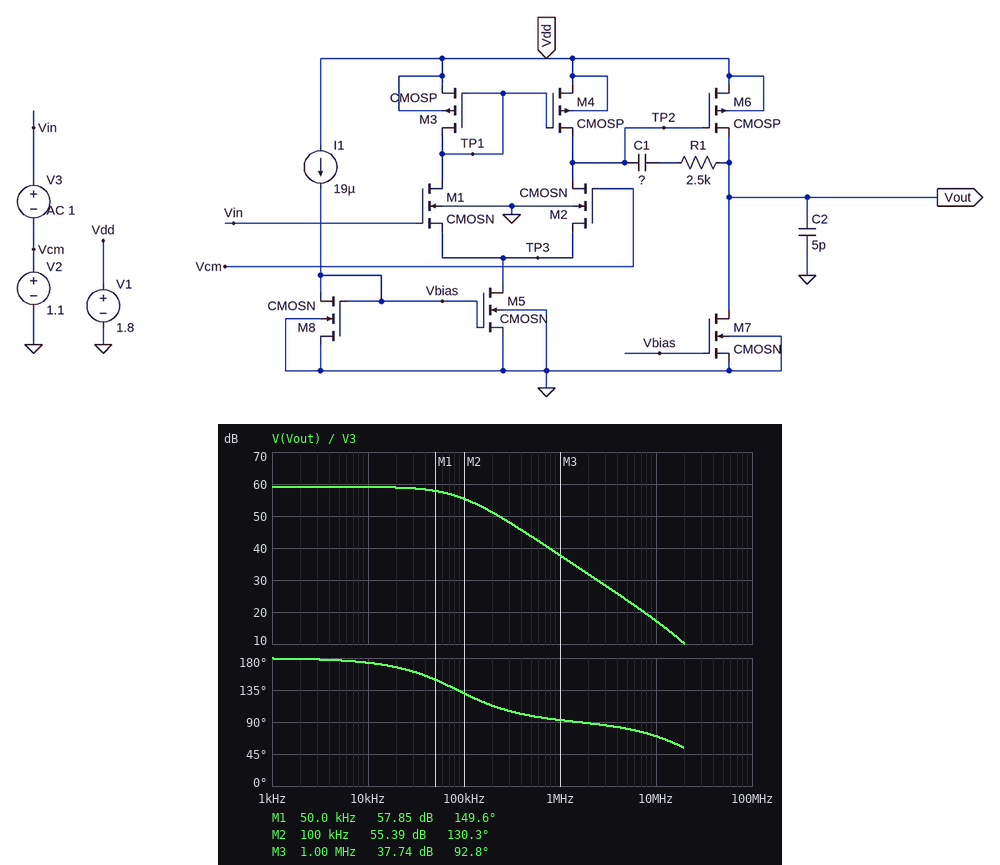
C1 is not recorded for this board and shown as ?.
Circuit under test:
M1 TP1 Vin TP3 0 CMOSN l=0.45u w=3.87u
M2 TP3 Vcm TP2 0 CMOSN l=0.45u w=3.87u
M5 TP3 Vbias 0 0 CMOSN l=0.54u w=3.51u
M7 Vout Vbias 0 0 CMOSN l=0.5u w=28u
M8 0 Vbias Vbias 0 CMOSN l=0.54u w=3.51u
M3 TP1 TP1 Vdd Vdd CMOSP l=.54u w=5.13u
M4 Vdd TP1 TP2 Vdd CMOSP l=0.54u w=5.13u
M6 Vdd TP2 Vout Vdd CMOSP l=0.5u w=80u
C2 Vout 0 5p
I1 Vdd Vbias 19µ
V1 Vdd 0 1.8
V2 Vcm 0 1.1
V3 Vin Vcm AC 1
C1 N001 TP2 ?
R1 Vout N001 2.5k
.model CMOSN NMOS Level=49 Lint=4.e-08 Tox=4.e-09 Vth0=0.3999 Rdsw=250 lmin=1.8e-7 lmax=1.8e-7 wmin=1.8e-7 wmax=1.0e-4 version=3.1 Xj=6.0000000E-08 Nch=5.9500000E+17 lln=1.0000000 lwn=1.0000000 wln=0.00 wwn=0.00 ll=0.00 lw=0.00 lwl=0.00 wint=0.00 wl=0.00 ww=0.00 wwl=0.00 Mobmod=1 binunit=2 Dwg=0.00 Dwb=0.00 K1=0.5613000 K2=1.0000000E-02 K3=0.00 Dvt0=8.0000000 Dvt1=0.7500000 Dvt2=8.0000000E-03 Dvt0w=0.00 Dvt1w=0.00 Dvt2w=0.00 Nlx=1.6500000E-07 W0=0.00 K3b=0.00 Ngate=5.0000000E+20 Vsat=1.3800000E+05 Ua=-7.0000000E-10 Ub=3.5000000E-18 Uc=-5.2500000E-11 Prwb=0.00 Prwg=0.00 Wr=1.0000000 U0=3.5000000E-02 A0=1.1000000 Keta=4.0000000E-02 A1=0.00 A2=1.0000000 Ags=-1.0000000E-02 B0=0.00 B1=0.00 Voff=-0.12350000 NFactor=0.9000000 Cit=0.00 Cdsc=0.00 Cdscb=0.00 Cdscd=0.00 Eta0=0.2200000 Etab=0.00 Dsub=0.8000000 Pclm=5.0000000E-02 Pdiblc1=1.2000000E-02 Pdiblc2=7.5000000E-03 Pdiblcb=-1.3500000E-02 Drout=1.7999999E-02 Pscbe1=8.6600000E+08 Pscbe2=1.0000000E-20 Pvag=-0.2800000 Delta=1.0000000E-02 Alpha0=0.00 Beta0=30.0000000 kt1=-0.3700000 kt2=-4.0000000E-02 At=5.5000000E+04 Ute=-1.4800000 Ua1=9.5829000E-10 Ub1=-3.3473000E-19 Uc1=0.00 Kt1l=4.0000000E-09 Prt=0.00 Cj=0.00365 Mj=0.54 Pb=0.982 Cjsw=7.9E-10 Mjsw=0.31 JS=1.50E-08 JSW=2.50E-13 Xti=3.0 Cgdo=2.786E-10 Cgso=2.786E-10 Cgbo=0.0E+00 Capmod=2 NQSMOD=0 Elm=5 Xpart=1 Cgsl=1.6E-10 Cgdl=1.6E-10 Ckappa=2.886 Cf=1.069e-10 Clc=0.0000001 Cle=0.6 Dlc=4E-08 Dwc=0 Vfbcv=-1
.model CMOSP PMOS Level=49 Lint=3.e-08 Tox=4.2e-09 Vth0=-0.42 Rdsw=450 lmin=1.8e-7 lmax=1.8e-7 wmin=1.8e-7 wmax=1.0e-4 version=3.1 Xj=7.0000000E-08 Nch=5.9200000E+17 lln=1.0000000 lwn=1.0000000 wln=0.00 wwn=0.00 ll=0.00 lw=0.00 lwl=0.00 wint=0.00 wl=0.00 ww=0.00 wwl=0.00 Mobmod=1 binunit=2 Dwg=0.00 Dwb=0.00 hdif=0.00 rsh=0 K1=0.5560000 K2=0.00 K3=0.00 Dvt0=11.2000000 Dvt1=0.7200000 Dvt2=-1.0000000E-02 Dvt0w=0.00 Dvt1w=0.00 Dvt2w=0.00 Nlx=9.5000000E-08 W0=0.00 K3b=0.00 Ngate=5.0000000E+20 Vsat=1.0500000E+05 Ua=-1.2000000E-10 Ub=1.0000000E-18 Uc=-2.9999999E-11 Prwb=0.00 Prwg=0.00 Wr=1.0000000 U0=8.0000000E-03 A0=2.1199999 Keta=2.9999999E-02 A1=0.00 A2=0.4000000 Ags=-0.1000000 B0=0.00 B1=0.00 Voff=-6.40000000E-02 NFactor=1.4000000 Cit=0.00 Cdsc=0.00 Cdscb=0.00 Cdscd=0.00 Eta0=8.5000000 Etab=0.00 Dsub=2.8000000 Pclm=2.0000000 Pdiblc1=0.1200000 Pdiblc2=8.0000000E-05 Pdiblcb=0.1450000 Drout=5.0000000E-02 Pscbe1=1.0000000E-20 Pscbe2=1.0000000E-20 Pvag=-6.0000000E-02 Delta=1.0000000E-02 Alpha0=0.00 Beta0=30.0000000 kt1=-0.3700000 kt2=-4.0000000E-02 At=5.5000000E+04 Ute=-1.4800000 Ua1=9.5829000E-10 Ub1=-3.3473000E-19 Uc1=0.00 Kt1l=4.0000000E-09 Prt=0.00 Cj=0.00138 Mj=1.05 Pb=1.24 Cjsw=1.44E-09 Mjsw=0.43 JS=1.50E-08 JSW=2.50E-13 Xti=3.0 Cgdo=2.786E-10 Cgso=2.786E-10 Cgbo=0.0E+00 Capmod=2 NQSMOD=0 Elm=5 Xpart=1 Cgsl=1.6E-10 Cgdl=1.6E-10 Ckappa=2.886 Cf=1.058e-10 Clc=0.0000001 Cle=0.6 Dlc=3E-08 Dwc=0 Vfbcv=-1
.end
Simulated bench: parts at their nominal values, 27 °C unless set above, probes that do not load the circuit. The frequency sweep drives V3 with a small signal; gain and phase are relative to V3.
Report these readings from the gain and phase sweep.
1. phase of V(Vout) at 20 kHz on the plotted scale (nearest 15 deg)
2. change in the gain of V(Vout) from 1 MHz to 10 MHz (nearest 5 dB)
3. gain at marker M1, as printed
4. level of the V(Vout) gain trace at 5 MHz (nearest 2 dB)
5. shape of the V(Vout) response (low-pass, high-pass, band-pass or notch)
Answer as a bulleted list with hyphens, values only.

- 165 deg
- -20 dB
- 57.85 dB
- 24 dB
- low-pass
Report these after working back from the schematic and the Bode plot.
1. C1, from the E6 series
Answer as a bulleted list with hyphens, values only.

- 220 fF
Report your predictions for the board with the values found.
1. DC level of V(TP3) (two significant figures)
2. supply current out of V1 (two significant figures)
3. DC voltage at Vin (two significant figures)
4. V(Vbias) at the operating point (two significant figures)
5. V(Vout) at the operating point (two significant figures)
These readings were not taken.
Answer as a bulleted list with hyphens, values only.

- 430 mV
- 200 µA
- 1.1 V
- 610 mV
- 930 mV
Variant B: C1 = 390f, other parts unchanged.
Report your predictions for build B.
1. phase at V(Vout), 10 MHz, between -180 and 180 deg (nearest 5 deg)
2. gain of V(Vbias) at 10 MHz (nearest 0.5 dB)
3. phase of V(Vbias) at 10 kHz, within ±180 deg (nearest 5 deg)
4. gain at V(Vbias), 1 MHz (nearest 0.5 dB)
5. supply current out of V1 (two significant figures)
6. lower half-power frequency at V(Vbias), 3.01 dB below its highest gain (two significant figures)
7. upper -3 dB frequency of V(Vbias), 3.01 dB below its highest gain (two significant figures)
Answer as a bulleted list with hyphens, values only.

- 75 deg
- -34.5 dB
- -100 deg
- -34.0 dB
- 200 µA
- 53 kHz
- 38 MHz
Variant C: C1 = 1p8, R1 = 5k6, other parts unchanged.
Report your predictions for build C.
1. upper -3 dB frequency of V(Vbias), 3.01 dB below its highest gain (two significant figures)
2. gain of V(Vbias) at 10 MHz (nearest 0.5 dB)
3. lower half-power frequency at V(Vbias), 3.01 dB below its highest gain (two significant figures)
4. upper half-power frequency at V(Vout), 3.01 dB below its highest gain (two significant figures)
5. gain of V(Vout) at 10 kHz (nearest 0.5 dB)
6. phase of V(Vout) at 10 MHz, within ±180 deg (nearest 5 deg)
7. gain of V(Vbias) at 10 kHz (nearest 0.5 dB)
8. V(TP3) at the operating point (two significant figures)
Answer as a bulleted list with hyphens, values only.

- 160 MHz
- -45.0 dB
- 28 MHz
- 13 kHz
- 57.0 dB
- 105 deg
- -50.5 dB
- 430 mV
